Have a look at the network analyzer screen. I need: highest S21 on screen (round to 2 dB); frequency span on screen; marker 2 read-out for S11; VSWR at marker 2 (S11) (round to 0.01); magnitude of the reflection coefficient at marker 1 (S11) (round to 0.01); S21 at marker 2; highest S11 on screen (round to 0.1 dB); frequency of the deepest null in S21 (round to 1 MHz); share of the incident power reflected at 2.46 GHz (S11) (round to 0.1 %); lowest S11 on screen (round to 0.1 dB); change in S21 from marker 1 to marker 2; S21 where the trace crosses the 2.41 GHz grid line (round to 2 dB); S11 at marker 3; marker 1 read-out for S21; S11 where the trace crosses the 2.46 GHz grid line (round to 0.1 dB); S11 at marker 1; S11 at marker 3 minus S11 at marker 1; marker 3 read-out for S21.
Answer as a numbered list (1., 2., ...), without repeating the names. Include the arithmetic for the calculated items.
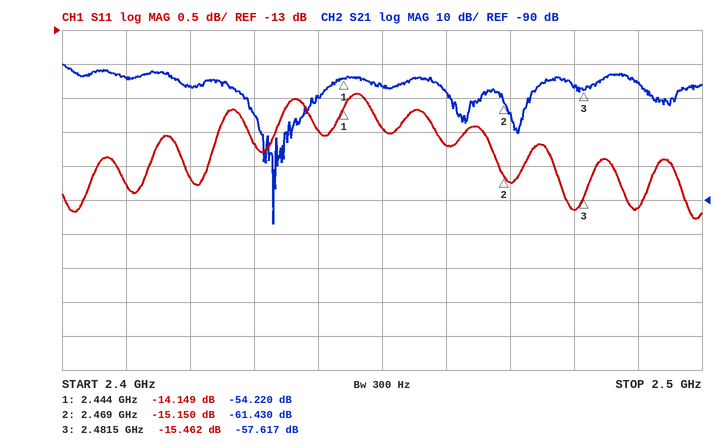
1. -50 dB
2. 100 MHz
3. -15.150 dB
4. (1 + 0.1748)/(1 − 0.1748) ≈ 1.42
5. 10^(-14.149/20) ≈ 0.20
6. -61.430 dB
7. -13.9 dB
8. 2.433 GHz
9. 10^(-14.7/10) ≈ 3.4 %
10. -15.8 dB
11. -61.43 − (-54.22) = -7.210 dB
12. -54 dB
13. -15.462 dB
14. -54.220 dB
15. -14.7 dB
16. -14.149 dB
17. -15.462 − (-14.149) = -1.313 dB
18. -57.617 dB
